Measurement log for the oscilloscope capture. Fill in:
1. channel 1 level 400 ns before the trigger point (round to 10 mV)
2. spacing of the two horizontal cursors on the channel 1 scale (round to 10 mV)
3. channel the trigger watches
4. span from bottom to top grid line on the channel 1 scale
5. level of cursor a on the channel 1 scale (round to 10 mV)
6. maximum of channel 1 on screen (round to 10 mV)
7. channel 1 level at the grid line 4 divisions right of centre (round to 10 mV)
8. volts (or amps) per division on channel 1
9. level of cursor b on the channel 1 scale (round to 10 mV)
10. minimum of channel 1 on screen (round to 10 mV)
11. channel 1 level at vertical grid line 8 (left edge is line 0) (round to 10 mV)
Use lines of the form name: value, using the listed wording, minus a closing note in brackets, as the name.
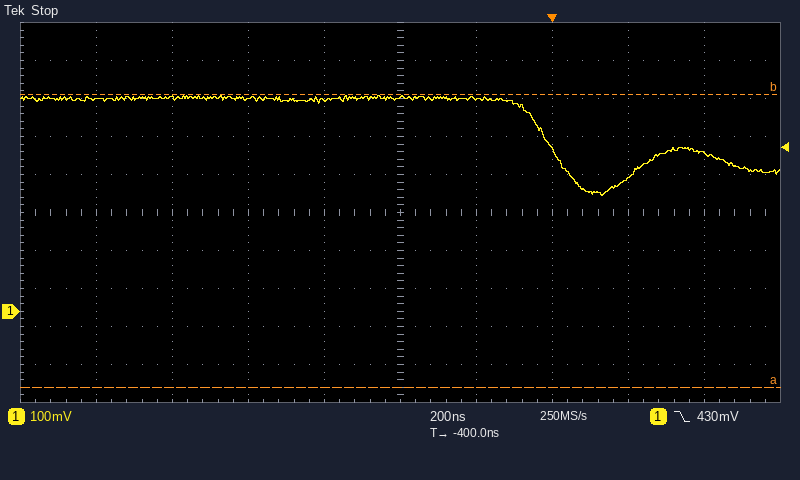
channel 1 level 400 ns before the trigger point: 560 mV
spacing of the two horizontal cursors on the channel 1 scale: 770 mV
channel the trigger watches: channel 1
span from bottom to top grid line on the channel 1 scale: 1 V
level of cursor a on the channel 1 scale: -200 mV
maximum of channel 1 on screen: 570 mV
channel 1 level at the grid line 4 divisions right of centre: 410 mV
volts (or amps) per division on channel 1: 100 mV
level of cursor b on the channel 1 scale: 570 mV
minimum of channel 1 on screen: 300 mV
channel 1 level at vertical grid line 8 (left edge is line 0): 350 mV
